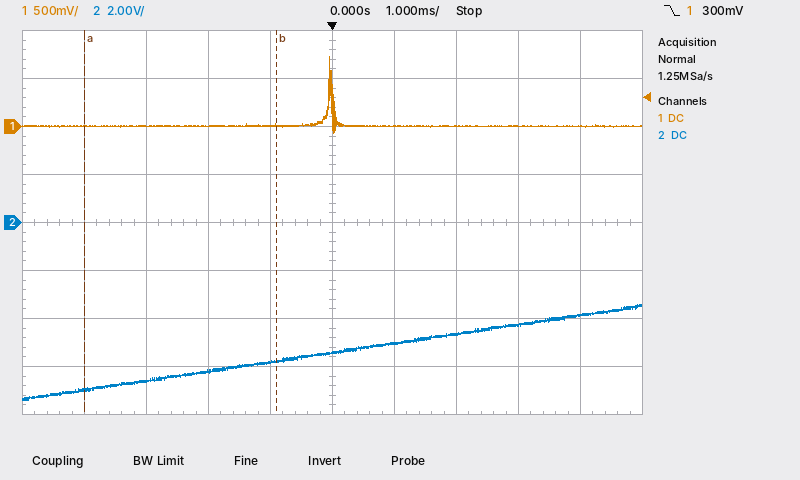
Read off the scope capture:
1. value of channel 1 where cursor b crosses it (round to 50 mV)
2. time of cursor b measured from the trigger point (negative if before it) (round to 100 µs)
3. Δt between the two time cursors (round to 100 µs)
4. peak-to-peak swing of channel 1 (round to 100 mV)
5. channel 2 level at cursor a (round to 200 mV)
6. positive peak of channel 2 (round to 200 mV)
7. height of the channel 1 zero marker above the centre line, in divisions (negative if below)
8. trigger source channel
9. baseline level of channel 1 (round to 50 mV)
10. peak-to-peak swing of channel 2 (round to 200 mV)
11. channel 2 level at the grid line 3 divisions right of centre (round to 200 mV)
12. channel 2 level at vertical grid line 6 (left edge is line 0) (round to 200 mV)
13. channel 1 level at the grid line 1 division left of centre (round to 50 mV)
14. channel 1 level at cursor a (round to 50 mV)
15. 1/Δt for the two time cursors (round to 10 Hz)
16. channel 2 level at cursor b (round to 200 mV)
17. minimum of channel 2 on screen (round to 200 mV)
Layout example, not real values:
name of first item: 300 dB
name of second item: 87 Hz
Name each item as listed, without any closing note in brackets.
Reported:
value of channel 1 where cursor b crosses it: 0 mV
time of cursor b measured from the trigger point (negative if before it): -900 µs
Δt between the two time cursors: 3.1 ms
peak-to-peak swing of channel 1: 800 mV
channel 2 level at cursor a: -7.0 V
positive peak of channel 2: -3.4 V
height of the channel 1 zero marker above the centre line, in divisions: +2.0 div
trigger source channel: channel 1
baseline level of channel 1: 0 mV
peak-to-peak swing of channel 2: 4.0 V
channel 2 level at the grid line 3 divisions right of centre: -4.2 V
channel 2 level at vertical grid line 6 (left edge is line 0): -5.0 V
channel 1 level at the grid line 1 division left of centre: 0 mV
channel 1 level at cursor a: 0 mV
1/Δt for the two time cursors: 320 Hz
channel 2 level at cursor b: -5.8 V
minimum of channel 2 on screen: -7.4 V
